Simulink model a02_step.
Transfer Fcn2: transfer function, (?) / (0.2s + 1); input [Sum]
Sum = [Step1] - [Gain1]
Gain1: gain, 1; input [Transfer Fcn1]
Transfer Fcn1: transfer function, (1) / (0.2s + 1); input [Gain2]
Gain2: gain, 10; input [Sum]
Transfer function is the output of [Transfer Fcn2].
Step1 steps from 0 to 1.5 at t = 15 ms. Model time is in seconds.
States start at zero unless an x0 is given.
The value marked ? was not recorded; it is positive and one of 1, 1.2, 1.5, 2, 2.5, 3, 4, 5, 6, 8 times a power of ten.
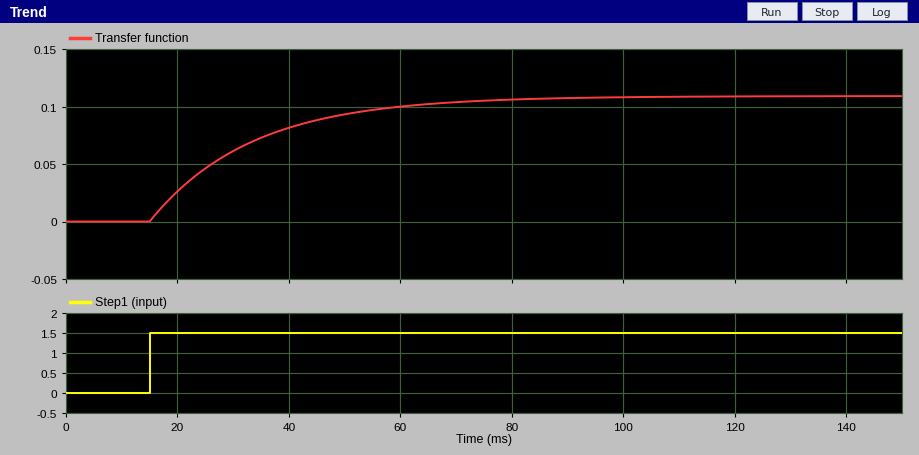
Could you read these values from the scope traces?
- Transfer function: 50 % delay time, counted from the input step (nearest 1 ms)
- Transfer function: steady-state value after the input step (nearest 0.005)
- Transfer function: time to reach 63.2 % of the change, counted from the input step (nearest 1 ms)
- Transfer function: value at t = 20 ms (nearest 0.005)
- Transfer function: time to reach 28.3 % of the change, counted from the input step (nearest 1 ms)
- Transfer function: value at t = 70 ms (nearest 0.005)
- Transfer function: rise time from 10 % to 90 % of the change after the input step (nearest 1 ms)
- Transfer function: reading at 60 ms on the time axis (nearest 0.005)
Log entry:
13 ms
0.110
18 ms
0.025
6 ms
0.105
40 ms
0.100
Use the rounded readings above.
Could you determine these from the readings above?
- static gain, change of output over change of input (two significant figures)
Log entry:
0.073
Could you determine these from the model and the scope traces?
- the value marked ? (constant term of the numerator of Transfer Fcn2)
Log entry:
0.8
